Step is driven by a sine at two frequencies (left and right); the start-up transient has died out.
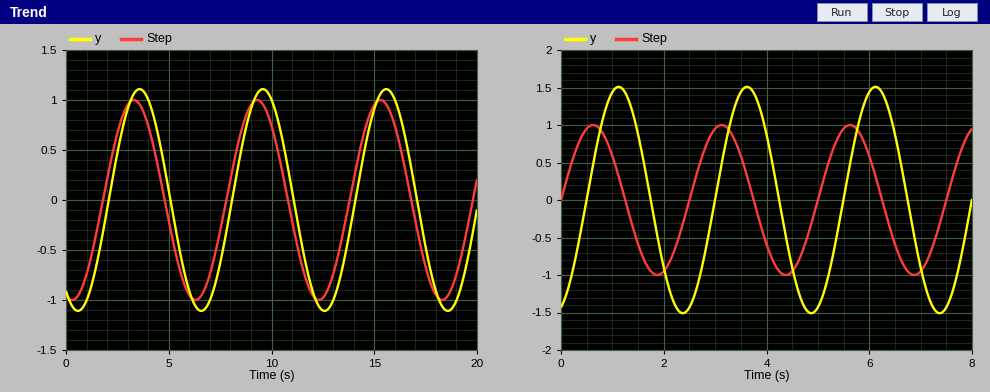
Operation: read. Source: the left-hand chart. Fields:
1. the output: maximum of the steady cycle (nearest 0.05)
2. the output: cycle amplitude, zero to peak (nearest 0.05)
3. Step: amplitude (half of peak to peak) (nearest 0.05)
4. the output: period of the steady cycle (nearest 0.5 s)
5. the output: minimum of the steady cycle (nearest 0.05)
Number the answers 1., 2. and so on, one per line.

1. 1.10
2. 1.10
3. 1.00
4. 6.0 s
5. -1.10
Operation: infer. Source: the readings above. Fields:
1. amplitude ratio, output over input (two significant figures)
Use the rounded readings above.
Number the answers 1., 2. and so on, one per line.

1. 1.1
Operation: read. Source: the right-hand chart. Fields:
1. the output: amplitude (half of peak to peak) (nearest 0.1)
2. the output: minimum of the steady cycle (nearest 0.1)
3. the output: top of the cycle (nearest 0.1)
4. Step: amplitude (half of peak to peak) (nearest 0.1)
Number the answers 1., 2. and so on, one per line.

1. 1.5
2. -1.5
3. 1.5
4. 1.0
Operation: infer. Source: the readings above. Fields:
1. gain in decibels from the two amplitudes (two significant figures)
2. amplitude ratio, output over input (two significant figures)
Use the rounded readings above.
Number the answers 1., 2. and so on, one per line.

1. 3.5 dB
2. 1.5
